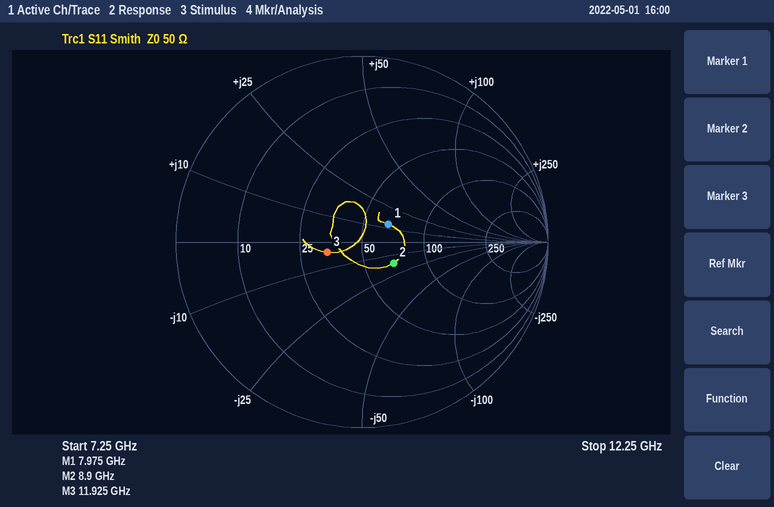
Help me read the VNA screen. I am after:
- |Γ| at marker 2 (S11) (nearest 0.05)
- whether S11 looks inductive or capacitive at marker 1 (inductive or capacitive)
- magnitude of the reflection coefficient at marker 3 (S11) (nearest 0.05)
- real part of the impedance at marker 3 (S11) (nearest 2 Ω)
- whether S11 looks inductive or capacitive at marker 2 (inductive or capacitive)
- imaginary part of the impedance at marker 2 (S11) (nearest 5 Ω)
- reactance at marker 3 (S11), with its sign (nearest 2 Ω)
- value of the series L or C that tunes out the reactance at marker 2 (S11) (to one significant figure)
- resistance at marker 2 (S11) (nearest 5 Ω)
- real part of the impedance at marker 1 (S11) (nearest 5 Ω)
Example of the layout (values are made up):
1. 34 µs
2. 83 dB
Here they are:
1. 0.20
2. inductive
3. 0.20
4. 34 Ω
5. capacitive
6. -15 Ω
7. -4 Ω
8. 300 pH
9. 70 Ω
10. 65 Ω
